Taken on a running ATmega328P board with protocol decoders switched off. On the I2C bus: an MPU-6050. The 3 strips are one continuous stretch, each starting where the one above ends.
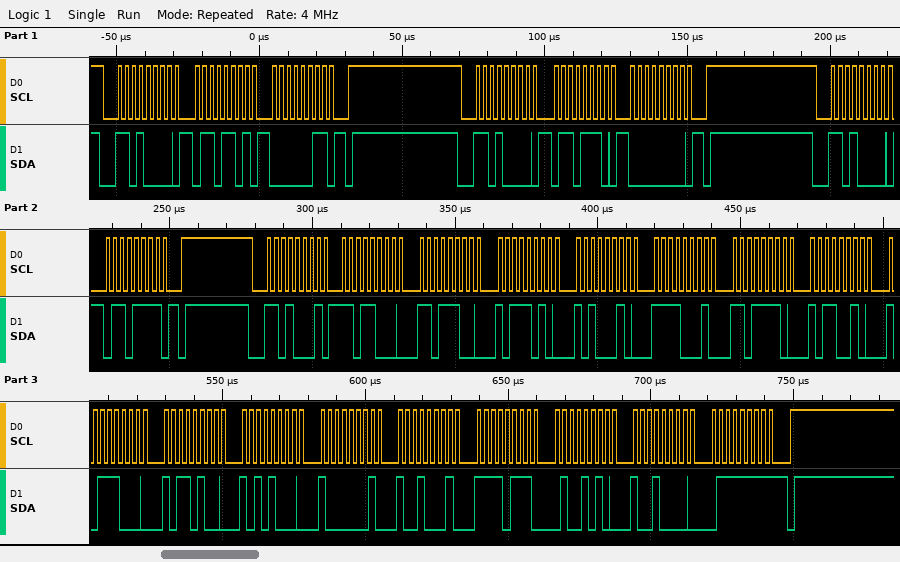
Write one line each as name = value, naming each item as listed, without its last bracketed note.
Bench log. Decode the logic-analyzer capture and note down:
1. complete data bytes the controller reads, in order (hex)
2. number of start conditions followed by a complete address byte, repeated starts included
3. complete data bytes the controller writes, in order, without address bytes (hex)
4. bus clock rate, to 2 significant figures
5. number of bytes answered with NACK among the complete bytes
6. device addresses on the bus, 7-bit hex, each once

complete data bytes the controller reads, in order = D8 DC BA A2 F1 DE B2 B8 B4 A8 81 91 F7 4A 90 7F
number of start conditions followed by a complete address byte, repeated starts included = 4
complete data bytes the controller writes, in order, without address bytes = 6D 03 6E 00 6F
bus clock rate, to 2 significant figures = 400 kHz
number of bytes answered with NACK among the complete bytes = 1
device addresses on the bus, 7-bit hex, each once = 0x68
